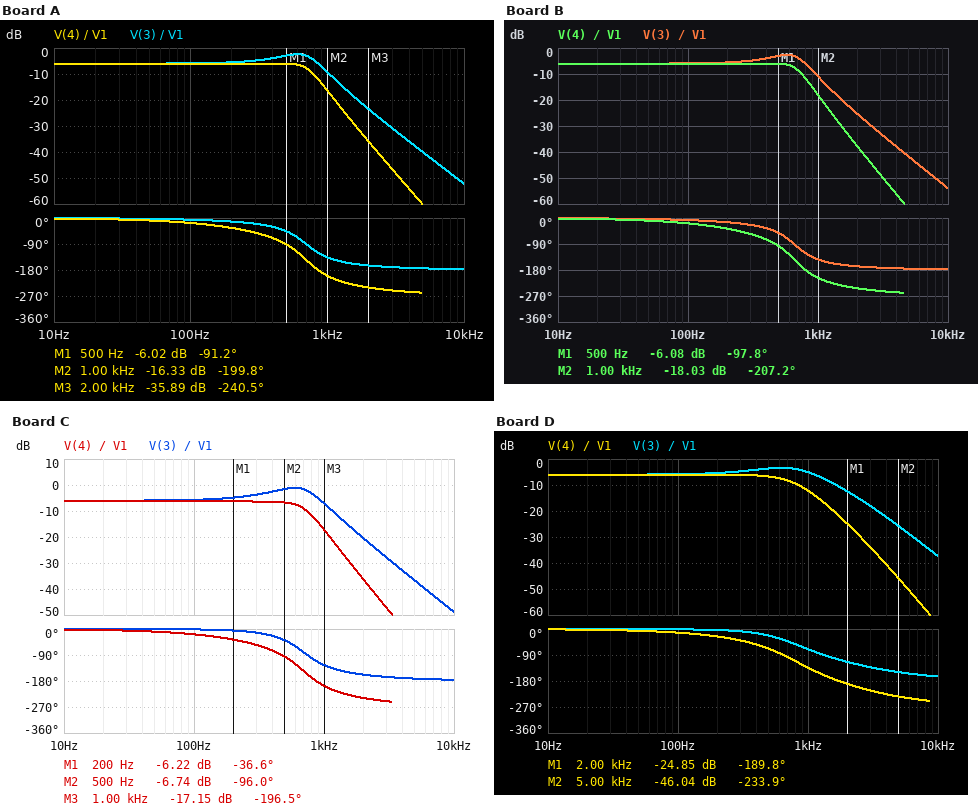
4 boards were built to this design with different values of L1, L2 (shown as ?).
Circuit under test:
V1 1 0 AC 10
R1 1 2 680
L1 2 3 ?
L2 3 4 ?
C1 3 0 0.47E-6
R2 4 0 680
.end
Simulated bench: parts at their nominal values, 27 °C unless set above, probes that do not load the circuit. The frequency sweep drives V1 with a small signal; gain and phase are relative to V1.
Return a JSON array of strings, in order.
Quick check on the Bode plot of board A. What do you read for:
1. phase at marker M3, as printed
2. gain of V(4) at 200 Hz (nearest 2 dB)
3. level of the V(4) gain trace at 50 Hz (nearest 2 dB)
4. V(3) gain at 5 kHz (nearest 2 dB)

["-240.5 deg", "-6 dB", "-6 dB", "-40 dB"]
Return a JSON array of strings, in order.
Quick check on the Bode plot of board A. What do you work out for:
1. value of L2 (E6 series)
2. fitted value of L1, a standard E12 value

["220 mH", "220 mH"]
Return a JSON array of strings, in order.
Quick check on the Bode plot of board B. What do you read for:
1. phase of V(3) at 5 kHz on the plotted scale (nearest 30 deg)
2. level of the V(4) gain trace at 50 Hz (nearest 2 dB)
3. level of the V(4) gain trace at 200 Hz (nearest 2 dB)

["-180 deg", "-6 dB", "-6 dB"]
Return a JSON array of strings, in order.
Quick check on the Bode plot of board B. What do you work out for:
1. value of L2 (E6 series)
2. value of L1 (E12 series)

["220 mH", "270 mH"]
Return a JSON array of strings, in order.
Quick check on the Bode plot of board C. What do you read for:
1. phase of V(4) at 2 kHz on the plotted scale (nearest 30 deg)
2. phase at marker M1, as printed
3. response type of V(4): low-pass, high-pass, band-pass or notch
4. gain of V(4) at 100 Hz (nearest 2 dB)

["-240 deg", "-36.6 deg", "low-pass", "-6 dB"]
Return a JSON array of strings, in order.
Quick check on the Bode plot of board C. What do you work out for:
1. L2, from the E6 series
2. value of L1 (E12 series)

["330 mH", "150 mH"]
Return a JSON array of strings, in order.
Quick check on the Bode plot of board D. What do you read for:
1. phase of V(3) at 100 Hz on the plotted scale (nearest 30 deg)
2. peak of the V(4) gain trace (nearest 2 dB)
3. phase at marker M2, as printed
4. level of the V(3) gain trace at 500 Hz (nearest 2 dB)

["0 deg", "-6 dB", "-233.9 deg", "-4 dB"]
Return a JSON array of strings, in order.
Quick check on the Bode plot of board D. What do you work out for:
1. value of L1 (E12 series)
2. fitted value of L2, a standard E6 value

["39 mH", "220 mH"]
